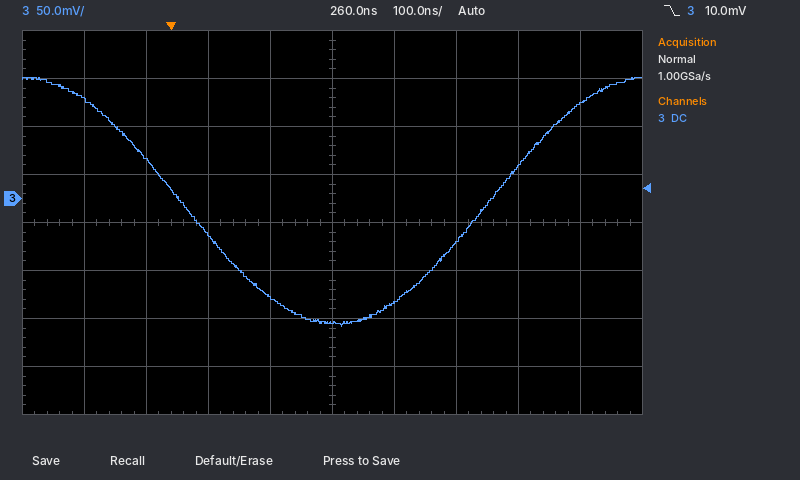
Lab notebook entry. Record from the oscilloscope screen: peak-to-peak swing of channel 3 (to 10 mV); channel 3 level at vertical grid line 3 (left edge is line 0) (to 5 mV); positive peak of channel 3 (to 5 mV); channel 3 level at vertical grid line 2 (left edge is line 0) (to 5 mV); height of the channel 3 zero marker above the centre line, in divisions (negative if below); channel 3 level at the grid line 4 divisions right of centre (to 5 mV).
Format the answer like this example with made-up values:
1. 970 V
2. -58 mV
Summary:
1. 260 mV
2. -40 mV
3. 125 mV
4. 40 mV
5. +0.5 div
6. 100 mV
